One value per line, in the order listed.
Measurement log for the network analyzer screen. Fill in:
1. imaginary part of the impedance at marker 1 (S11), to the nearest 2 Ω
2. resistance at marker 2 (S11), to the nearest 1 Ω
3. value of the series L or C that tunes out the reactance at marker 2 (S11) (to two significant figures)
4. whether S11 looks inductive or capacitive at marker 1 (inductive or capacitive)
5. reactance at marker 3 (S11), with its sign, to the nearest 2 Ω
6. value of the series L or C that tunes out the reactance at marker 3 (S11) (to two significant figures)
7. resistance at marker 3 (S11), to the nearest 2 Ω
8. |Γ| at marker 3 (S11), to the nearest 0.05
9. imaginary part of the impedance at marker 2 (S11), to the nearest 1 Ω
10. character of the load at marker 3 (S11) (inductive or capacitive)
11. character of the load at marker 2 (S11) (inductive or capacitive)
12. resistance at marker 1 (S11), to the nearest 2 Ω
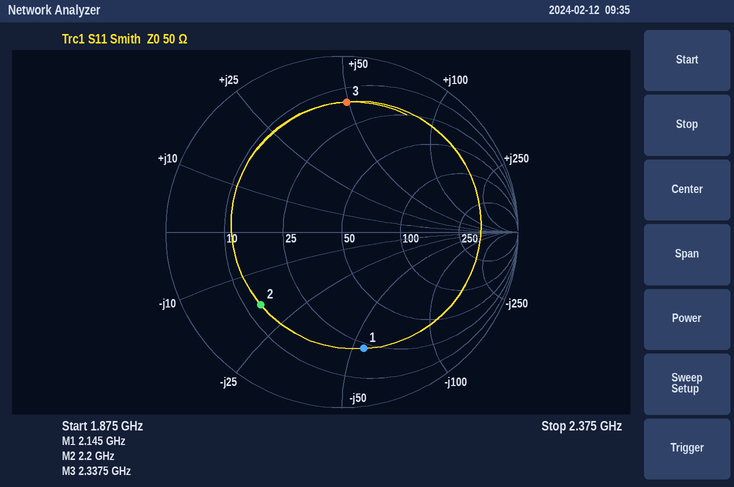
-54 Ω
13 Ω
1.3 nH
capacitive
+50 Ω
1.4 pF
16 Ω
0.75
-18 Ω
inductive
capacitive
22 Ω
